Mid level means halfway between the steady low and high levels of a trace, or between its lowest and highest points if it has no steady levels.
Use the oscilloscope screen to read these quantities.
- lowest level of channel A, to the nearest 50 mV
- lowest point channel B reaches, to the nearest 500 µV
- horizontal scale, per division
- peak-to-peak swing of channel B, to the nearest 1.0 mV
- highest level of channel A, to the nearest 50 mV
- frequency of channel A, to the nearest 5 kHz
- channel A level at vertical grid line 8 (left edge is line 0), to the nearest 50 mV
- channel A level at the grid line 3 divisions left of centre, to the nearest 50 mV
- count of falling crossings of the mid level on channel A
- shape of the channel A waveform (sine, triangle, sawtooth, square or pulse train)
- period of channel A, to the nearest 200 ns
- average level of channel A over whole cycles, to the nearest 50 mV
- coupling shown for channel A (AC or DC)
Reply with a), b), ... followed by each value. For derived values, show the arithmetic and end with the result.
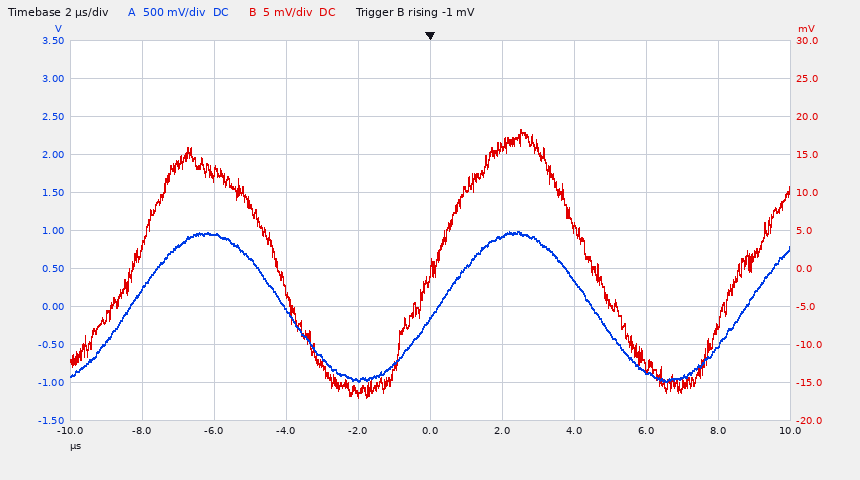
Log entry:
a) -1.00 V
b) -17.0 mV
c) 2 µs
d) 35.0 mV
e) 1.00 V
f) 1 / 8.6 µs ≈ 116 kHz, so 115 kHz to the nearest 5 kHz
g) -850 mV
h) 950 mV
i) 2
j) sine
k) 8.6 µs
l) (1.00 V + (-1.00 V)) / 2 ≈ 0 mV
m) DC
